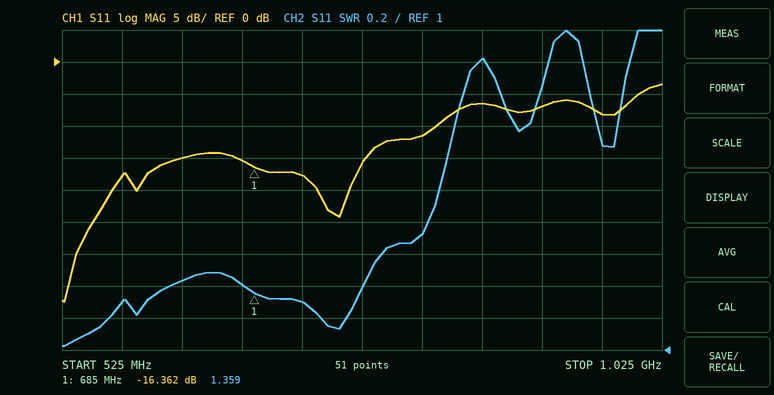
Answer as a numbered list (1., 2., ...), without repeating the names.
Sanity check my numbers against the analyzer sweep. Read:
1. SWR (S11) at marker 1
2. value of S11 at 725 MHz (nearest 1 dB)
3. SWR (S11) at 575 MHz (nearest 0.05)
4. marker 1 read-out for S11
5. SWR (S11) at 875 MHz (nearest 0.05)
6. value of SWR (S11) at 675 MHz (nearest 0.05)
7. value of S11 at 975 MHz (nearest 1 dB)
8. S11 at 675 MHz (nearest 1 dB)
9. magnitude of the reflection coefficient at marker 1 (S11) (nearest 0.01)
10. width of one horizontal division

1. 1.359
2. -18 dB
3. 1.30
4. -16.362 dB
5. 2.80
6. 1.40
7. -8 dB
8. -15 dB
9. 0.15
10. 50 MHz
